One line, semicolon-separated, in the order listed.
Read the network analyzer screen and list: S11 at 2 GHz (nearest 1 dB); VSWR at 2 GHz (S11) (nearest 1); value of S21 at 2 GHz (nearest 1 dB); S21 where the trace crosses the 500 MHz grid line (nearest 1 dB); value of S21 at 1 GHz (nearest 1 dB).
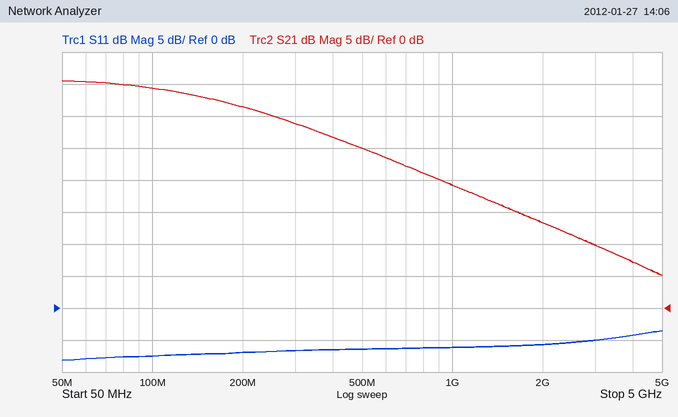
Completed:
-6 dB; 3; 13 dB; 25 dB; 19 dB
